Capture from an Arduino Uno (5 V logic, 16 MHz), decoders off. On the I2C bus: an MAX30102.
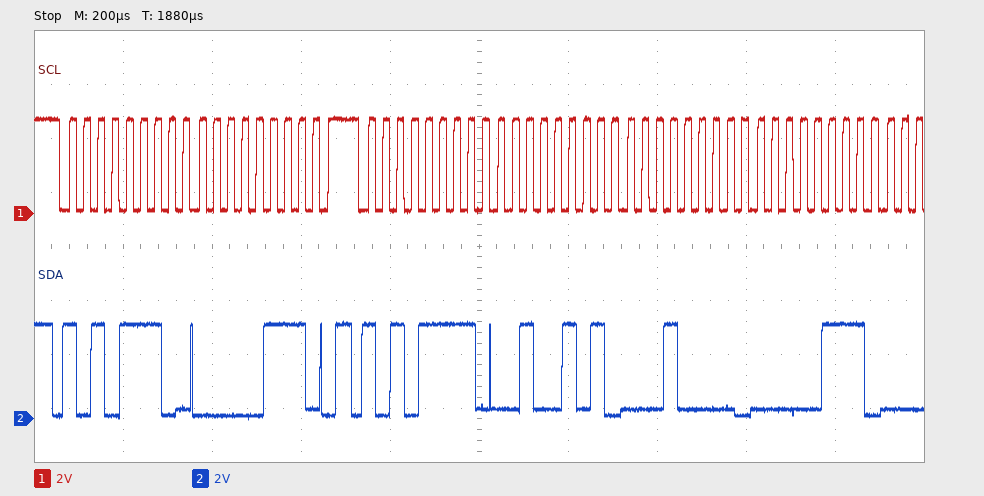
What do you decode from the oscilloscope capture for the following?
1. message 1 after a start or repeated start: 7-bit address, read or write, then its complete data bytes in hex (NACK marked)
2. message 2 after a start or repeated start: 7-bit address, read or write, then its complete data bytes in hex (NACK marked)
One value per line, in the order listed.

0x57 write: 07
0x57 read: 25 10 07
